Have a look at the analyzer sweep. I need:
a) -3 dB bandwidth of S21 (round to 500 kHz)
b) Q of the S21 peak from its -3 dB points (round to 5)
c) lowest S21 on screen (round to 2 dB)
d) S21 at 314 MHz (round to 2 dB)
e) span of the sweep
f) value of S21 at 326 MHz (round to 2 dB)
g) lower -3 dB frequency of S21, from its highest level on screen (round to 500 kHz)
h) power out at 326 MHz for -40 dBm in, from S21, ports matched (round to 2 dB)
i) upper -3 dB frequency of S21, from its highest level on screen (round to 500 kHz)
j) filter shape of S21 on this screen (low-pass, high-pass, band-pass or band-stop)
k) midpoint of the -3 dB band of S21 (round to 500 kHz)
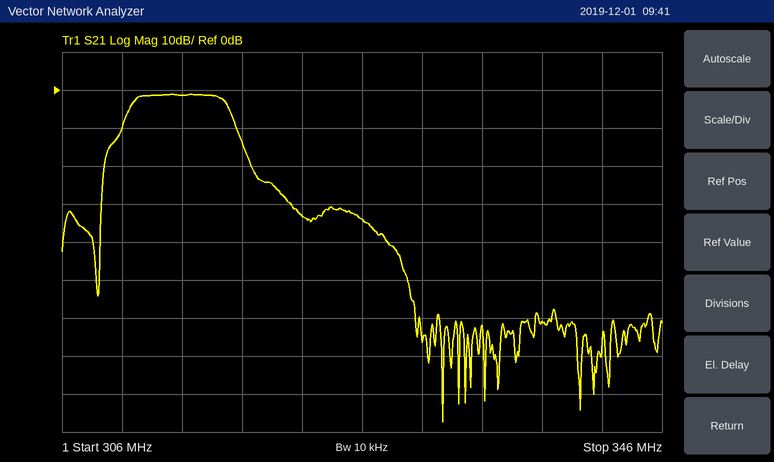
6.5 MHz
50
-88 dB
-2 dB
40 MHz
-34 dB
310.5 MHz
-74 dBm
317.0 MHz
band-pass
314.0 MHz
